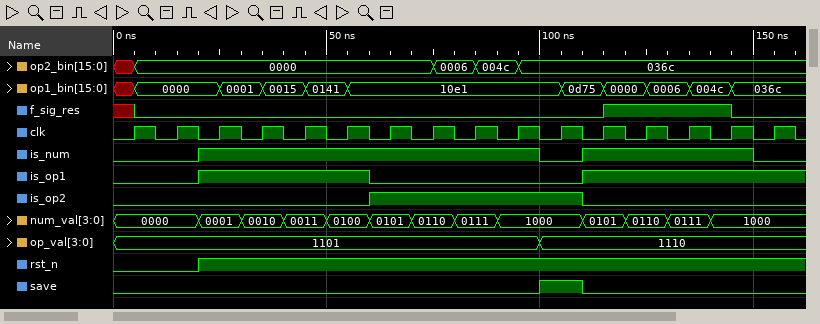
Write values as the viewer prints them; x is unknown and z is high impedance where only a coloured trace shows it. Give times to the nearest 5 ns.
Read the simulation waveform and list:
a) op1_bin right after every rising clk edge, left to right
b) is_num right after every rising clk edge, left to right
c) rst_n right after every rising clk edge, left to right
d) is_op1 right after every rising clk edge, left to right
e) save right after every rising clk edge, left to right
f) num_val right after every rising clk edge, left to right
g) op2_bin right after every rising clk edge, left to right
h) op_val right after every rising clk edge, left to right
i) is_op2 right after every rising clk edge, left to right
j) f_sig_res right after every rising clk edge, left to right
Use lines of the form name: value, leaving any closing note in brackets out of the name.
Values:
op1_bin right after every rising clk edge, left to right: 0000, 0000, 0001, 0015, 0141, 10e1, 10e1, 10e1, 10e1, 10e1, 0d75, 0000, 0006, 004c, 036c, 036c
is_num right after every rising clk edge, left to right: 0 0 1 1 1 1 1 1 1 1 0 1 1 1 1 0
rst_n right after every rising clk edge, left to right: 0 0 1 1 1 1 1 1 1 1 1 1 1 1 1 1
is_op1 right after every rising clk edge, left to right: 0 0 1 1 1 1 0 0 0 0 0 1 1 1 1 1
save right after every rising clk edge, left to right: 0 0 0 0 0 0 0 0 0 0 1 0 0 0 0 0
num_val right after every rising clk edge, left to right: 0000, 0000, 0001, 0010, 0011, 0100, 0101, 0110, 0111, 1000, 1000, 0101, 0110, 0111, 1000, 1000
op2_bin right after every rising clk edge, left to right: 0000, 0000, 0000, 0000, 0000, 0000, 0000, 0006, 004c, 036c, 036c, 036c, 036c, 036c, 036c, 036c
op_val right after every rising clk edge, left to right: 1101, 1101, 1101, 1101, 1101, 1101, 1101, 1101, 1101, 1101, 1110, 1110, 1110, 1110, 1110, 1110
is_op2 right after every rising clk edge, left to right: 0 0 0 0 0 0 1 1 1 1 1 0 0 0 0 0
f_sig_res right after every rising clk edge, left to right: 0 0 0 0 0 0 0 0 0 0 0 1 1 1 0 0
